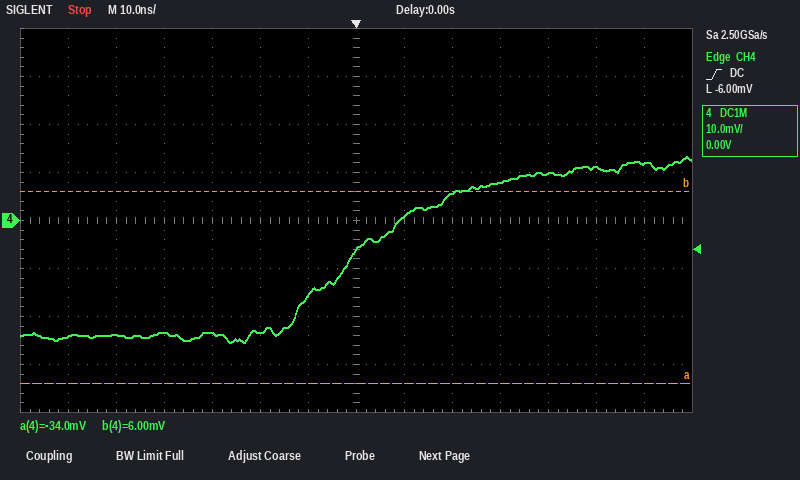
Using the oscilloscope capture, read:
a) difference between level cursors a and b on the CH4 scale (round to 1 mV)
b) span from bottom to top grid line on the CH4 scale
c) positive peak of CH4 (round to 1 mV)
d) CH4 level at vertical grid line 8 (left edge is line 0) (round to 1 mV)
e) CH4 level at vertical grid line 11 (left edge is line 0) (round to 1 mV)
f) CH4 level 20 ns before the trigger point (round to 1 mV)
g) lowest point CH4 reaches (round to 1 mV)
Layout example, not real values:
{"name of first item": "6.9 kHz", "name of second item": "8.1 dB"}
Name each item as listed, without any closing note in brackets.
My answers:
{"difference between level cursors a and b on the CH4 scale": "40 mV", "span from bottom to top grid line on the CH4 scale": "80 mV", "positive peak of CH4": "13 mV", "CH4 level at vertical grid line 8 (left edge is line 0)": "1 mV", "CH4 level at vertical grid line 11 (left edge is line 0)": "10 mV", "CH4 level 20 ns before the trigger point": "-23 mV", "lowest point CH4 reaches": "-25 mV"}
